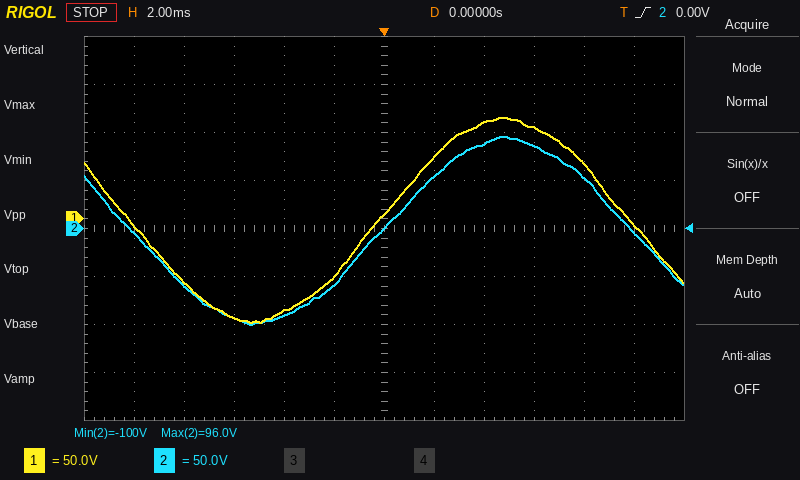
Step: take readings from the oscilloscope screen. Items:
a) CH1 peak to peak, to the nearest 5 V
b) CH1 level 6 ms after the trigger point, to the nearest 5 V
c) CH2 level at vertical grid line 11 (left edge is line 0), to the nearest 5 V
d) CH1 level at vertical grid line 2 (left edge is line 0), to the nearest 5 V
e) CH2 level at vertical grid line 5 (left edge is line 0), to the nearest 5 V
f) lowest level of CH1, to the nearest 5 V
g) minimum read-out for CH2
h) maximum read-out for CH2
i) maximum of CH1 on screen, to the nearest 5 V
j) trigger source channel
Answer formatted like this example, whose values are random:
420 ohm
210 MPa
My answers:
215 V
95 V
-5 V
-65 V
-60 V
-110 V
-100 V
96.0 V
105 V
CH2
